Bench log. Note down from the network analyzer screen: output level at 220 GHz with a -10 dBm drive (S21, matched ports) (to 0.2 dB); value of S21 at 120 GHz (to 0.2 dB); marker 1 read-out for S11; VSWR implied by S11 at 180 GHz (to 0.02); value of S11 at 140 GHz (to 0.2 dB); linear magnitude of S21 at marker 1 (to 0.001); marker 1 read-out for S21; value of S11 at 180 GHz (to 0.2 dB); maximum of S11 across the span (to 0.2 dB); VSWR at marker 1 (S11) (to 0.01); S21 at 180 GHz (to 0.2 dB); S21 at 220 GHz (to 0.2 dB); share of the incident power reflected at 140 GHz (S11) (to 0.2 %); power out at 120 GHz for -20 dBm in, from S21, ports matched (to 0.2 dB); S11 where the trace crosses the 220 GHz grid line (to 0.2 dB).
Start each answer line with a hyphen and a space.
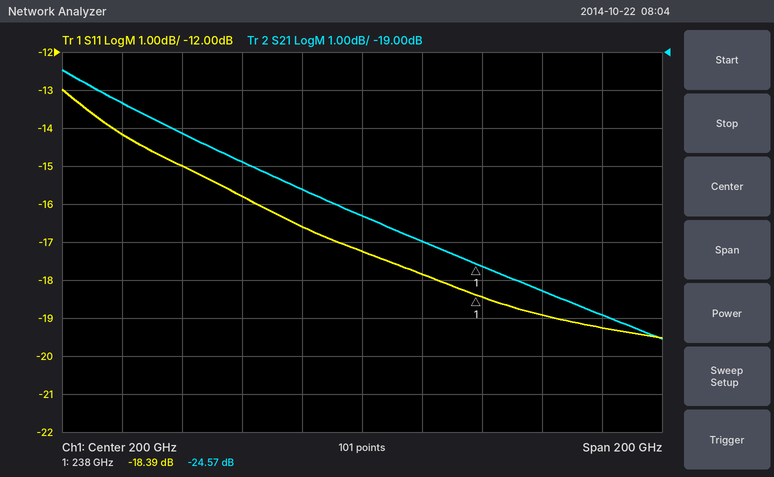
- -34.0 dBm
- -20.4 dB
- -18.39 dB
- 1.34
- -15.0 dB
- 0.059
- -24.57 dB
- -16.6 dB
- -13.0 dB
- 1.27
- -22.6 dB
- -24.0 dB
- 3.2 %
- -40.4 dBm
- -17.8 dB
